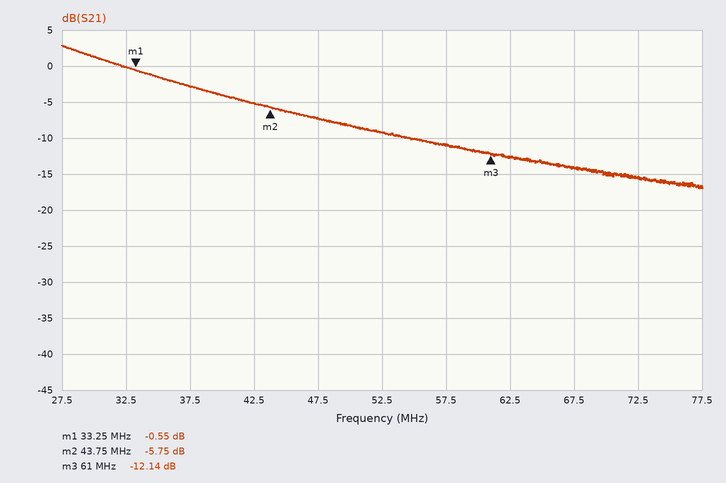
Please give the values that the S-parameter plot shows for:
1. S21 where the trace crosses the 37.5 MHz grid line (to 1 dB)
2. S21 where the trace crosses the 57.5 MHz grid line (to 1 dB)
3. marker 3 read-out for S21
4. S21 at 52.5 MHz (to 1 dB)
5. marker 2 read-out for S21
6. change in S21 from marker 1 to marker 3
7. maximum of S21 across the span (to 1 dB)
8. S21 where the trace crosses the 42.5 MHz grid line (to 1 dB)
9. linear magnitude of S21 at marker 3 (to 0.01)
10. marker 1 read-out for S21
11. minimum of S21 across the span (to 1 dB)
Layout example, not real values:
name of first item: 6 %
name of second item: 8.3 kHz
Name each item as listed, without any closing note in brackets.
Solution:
S21 where the trace crosses the 37.5 MHz grid line: -3 dB
S21 where the trace crosses the 57.5 MHz grid line: -11 dB
marker 3 read-out for S21: -12.14 dB
S21 at 52.5 MHz: -9 dB
marker 2 read-out for S21: -5.75 dB
change in S21 from marker 1 to marker 3: -11.59 dB
maximum of S21 across the span: 3 dB
S21 where the trace crosses the 42.5 MHz grid line: -5 dB
linear magnitude of S21 at marker 3: 0.25
marker 1 read-out for S21: -0.55 dB
minimum of S21 across the span: -17 dB
